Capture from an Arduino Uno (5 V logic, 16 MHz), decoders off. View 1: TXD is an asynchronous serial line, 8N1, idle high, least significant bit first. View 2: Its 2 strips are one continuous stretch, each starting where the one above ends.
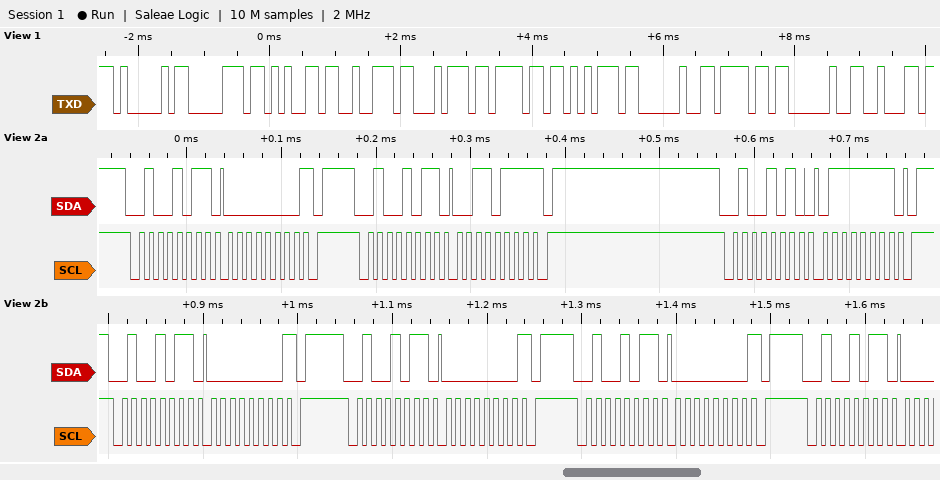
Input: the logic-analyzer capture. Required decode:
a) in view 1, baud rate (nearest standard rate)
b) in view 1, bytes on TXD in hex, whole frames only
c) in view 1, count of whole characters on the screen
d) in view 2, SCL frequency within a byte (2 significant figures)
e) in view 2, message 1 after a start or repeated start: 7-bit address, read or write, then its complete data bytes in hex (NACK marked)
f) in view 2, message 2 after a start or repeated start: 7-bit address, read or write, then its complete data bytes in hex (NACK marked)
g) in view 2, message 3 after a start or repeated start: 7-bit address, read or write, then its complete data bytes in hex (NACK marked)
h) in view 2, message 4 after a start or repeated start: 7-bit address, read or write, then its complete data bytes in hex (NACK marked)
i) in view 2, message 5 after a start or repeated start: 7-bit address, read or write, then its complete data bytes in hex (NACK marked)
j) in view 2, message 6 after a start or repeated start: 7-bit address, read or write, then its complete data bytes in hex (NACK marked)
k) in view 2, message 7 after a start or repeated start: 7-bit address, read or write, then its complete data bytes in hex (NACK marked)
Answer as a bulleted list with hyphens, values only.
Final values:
- 9600 baud
- 41 70 65 72 74 6F 75 20 6F 20 62
- 11
- 100 kHz
- 0x25 read: 00 NACK
- 0x25 read: 37 NACK
- 0x25 write: 7F
- 0x25 read: 00 NACK
- 0x25 read: 00 NACK
- 0x25 read: 00 NACK
- 0x25 read
